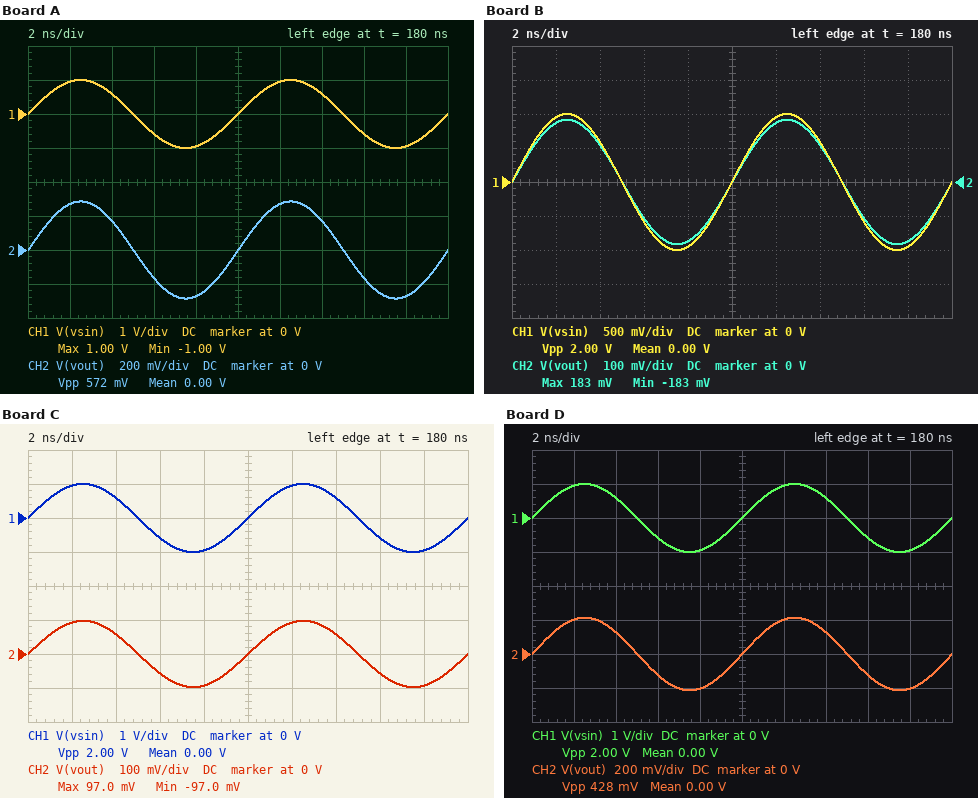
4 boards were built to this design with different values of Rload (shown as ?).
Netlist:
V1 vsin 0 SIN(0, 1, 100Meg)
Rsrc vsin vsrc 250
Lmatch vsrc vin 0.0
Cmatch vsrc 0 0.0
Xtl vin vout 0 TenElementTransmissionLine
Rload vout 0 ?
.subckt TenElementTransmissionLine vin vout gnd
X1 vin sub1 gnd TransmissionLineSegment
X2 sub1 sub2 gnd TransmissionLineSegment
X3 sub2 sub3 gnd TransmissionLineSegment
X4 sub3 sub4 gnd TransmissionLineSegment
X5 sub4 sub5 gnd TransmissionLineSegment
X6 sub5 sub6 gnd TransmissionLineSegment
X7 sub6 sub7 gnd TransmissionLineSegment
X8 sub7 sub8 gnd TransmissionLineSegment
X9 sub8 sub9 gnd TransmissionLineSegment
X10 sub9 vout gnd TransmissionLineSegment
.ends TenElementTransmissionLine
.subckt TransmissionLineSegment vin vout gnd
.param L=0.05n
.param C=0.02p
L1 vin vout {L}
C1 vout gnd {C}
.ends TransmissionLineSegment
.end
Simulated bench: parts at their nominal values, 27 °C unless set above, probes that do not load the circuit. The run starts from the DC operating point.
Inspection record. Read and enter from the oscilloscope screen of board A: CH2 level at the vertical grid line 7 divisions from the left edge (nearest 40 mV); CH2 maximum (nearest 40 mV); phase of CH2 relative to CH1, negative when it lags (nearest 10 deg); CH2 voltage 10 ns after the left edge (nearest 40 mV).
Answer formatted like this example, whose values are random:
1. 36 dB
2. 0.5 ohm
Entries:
1. 160 mV
2. 280 mV
3. 0 deg
4. 0 V
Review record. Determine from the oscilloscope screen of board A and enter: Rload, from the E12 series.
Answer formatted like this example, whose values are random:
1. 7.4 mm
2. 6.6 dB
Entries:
1. 100 Ω
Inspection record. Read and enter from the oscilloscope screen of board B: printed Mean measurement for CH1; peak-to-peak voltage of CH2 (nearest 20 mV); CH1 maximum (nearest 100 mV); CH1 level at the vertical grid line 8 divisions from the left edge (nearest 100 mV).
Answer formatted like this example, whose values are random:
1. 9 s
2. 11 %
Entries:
1. 0.00 V
2. 360 mV
3. 1.0 V
4. -600 mV
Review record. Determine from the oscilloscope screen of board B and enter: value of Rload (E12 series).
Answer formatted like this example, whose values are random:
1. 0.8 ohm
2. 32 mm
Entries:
1. 56 Ω
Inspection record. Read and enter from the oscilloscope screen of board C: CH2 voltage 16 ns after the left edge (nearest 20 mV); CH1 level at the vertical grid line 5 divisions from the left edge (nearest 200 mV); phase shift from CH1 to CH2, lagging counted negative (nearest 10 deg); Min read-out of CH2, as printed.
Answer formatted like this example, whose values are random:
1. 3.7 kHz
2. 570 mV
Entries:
1. -60 mV
2. 0 V
3. 0 deg
4. -97.0 mV
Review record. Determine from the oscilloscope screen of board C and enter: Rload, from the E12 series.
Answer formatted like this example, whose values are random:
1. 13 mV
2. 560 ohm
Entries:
1. 27 Ω
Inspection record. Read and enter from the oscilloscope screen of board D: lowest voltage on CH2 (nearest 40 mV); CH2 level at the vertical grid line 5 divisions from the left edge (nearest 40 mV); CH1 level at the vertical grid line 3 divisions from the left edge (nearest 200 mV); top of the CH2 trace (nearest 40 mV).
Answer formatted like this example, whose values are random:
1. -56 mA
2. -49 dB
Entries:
1. -200 mV
2. 0 V
3. -600 mV
4. 200 mV
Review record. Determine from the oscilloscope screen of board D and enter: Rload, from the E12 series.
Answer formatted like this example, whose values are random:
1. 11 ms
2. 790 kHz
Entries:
1. 68 Ω
